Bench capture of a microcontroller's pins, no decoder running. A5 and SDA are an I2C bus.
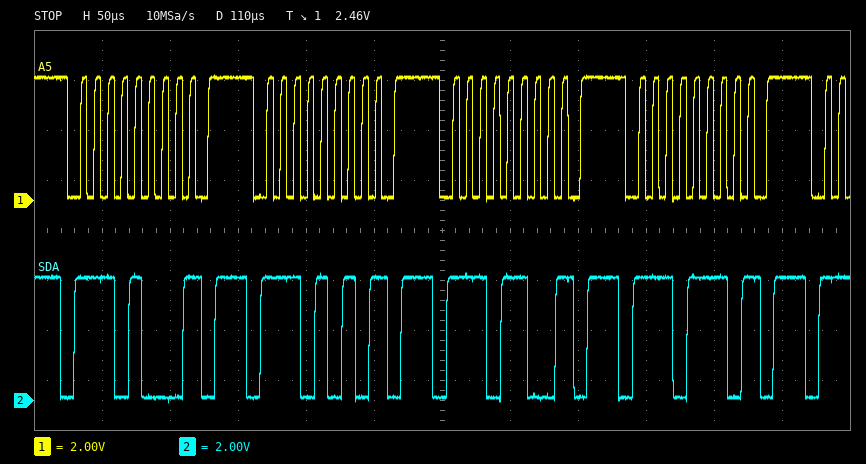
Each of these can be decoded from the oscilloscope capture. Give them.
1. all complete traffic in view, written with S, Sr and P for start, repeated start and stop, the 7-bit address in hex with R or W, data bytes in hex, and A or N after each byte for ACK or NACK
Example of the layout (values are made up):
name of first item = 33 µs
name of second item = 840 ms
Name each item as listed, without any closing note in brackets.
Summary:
all complete traffic in view, written with S, Sr and P for start, repeated start and stop, the 7-bit address in hex with R or W, data bytes in hex, and A or N after each byte for ACK or NACK = S 74W N P S 75W N P S 76W N P S 77W N P
